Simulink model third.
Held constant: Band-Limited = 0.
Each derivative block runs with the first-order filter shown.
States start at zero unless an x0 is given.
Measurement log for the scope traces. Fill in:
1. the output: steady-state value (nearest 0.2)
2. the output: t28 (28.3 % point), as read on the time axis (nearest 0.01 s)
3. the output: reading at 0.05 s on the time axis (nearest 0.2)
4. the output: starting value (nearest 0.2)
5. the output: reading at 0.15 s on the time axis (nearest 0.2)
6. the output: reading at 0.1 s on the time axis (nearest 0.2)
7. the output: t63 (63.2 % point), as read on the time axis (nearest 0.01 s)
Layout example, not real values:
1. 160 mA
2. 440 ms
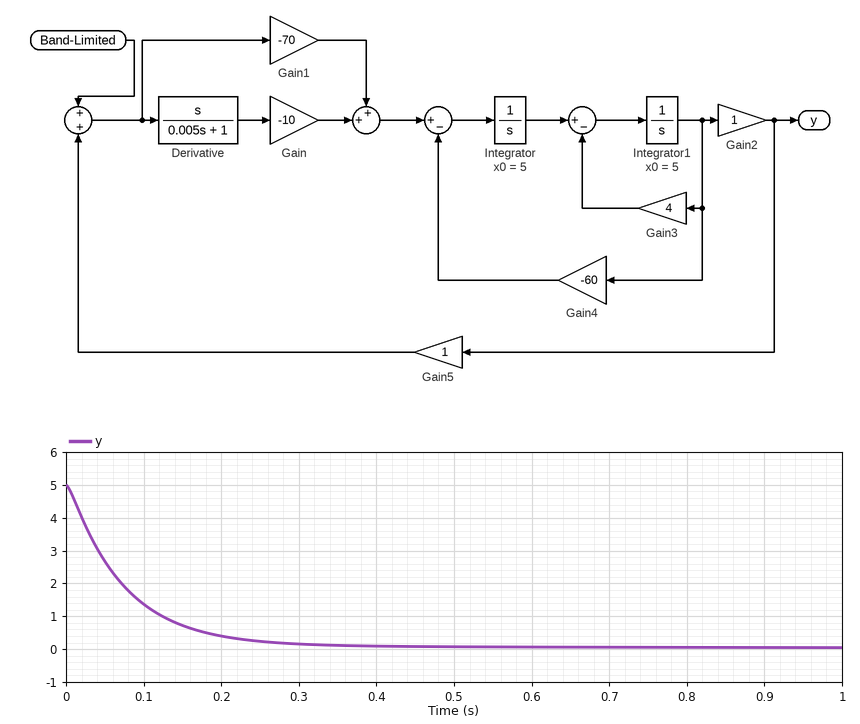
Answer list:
1. 0.0
2. 0.03 s
3. 2.6
4. 5.0
5. 0.8
6. 1.4
7. 0.08 s
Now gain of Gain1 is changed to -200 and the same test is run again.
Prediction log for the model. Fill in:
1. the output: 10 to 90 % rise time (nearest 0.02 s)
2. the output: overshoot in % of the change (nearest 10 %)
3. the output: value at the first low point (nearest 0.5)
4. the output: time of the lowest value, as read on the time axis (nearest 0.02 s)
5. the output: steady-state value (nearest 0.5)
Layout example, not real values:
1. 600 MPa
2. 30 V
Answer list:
1. 0.08 s
2. 20 %
3. -1.0
4. 0.20 s
5. 0.0
